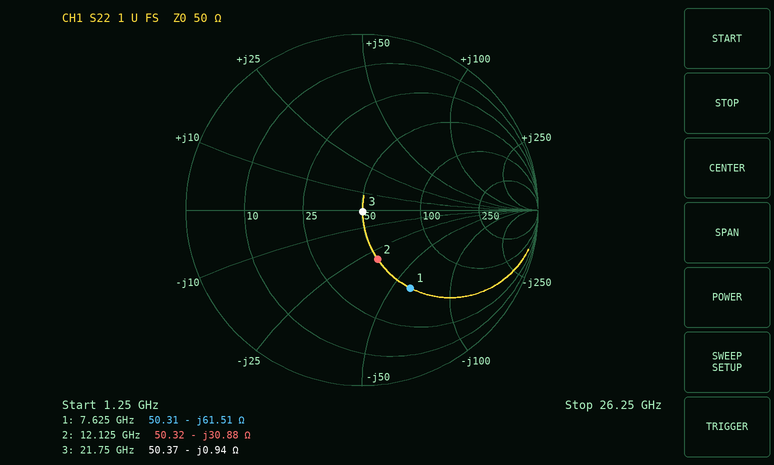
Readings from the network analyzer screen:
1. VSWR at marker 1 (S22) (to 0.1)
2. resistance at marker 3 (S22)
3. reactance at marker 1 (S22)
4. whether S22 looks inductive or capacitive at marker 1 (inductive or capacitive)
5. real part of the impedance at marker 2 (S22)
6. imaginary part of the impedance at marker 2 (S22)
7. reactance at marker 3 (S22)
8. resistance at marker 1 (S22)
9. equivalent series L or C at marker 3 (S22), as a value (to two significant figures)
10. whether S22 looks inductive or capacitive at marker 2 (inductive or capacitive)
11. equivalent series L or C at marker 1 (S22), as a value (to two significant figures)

3.2
50.37 Ω
-61.51 Ω
capacitive
50.32 Ω
-30.88 Ω
-0.94 Ω
50.31 Ω
7.8 pF
capacitive
340 fF
